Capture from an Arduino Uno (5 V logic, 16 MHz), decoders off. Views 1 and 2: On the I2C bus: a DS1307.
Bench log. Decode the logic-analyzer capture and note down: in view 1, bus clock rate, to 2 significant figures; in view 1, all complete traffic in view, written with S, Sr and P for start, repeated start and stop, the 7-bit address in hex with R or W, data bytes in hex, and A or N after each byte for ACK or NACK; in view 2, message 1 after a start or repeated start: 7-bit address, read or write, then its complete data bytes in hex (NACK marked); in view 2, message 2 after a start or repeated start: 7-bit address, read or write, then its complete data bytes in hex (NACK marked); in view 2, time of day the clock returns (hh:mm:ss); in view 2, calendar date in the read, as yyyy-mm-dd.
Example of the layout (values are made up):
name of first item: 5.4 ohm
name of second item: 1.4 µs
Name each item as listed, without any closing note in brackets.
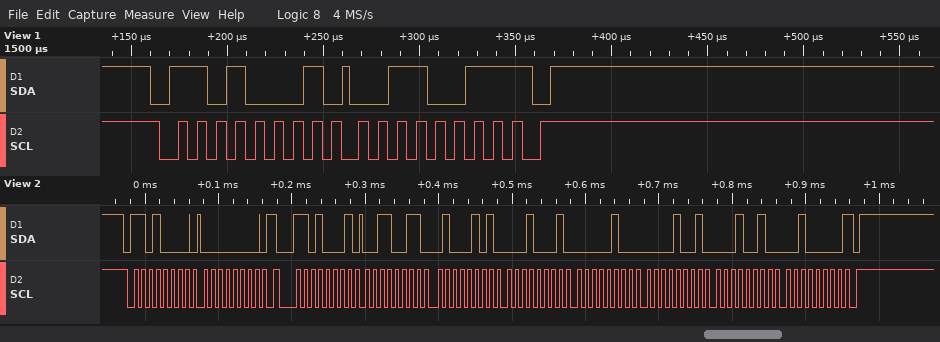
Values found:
in view 1, bus clock rate, to 2 significant figures: 100 kHz
in view 1, all complete traffic in view, written with S, Sr and P for start, repeated start and stop, the 7-bit address in hex with R or W, data bytes in hex, and A or N after each byte for ACK or NACK: S 68R A 33 N P
in view 2, message 1 after a start or repeated start: 7-bit address, read or write, then its complete data bytes in hex: 0x68 write: 00
in view 2, message 2 after a start or repeated start: 7-bit address, read or write, then its complete data bytes in hex: 0x68 read: 33 45 11 04 09 12 20 NACK
in view 2, time of day the clock returns: 11:45:33
in view 2, calendar date in the read, as yyyy-mm-dd: 2020-12-09
